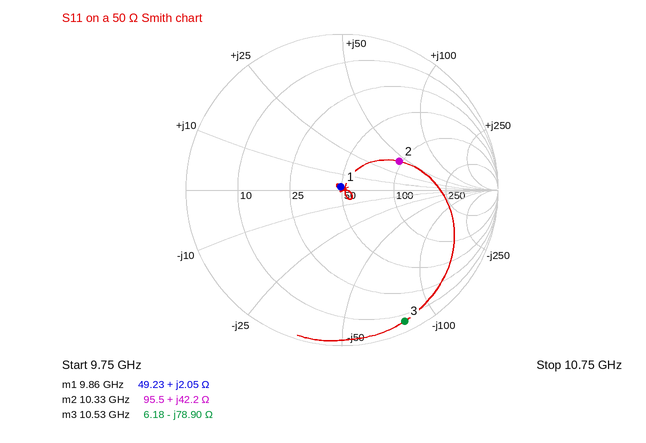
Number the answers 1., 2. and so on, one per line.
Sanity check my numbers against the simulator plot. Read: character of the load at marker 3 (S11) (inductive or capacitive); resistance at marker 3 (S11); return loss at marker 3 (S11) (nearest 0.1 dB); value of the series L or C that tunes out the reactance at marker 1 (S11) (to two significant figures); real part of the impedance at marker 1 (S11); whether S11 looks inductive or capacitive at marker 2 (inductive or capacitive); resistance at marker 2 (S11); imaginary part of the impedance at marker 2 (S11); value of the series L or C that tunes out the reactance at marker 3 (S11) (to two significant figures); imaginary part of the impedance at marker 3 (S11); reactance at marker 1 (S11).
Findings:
1. capacitive
2. 6.18 Ω
3. 0.6 dB
4. 7.9 pF
5. 49.23 Ω
6. inductive
7. 95.5 Ω
8. +42.2 Ω
9. 1.2 nH
10. -78.90 Ω
11. +2.05 Ω
